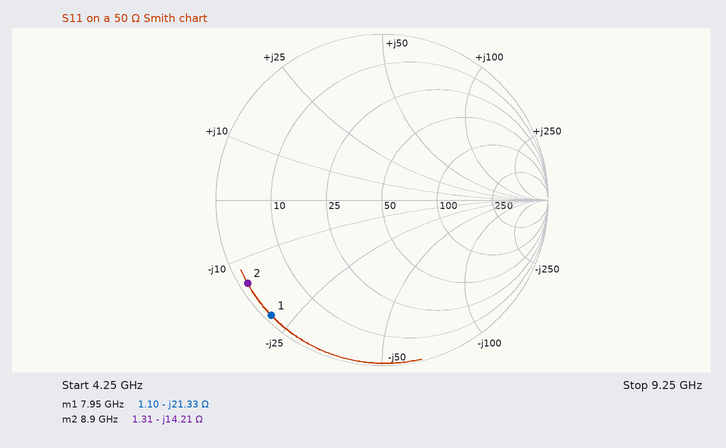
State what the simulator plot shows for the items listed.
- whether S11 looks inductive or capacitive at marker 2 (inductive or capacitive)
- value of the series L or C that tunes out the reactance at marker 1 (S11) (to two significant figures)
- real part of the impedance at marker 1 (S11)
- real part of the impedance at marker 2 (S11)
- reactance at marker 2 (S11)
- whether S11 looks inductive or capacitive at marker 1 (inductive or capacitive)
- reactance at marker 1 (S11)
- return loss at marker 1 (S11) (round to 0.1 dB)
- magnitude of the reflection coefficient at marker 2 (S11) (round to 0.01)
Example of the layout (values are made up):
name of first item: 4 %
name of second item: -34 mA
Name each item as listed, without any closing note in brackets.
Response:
whether S11 looks inductive or capacitive at marker 2: capacitive
value of the series L or C that tunes out the reactance at marker 1 (S11): 430 pH
real part of the impedance at marker 1: 1.10 Ω
real part of the impedance at marker 2: 1.31 Ω
reactance at marker 2: -14.21 Ω
whether S11 looks inductive or capacitive at marker 1: capacitive
reactance at marker 1: -21.33 Ω
return loss at marker 1 (S11): 0.3 dB
magnitude of the reflection coefficient at marker 2 (S11): 0.95
